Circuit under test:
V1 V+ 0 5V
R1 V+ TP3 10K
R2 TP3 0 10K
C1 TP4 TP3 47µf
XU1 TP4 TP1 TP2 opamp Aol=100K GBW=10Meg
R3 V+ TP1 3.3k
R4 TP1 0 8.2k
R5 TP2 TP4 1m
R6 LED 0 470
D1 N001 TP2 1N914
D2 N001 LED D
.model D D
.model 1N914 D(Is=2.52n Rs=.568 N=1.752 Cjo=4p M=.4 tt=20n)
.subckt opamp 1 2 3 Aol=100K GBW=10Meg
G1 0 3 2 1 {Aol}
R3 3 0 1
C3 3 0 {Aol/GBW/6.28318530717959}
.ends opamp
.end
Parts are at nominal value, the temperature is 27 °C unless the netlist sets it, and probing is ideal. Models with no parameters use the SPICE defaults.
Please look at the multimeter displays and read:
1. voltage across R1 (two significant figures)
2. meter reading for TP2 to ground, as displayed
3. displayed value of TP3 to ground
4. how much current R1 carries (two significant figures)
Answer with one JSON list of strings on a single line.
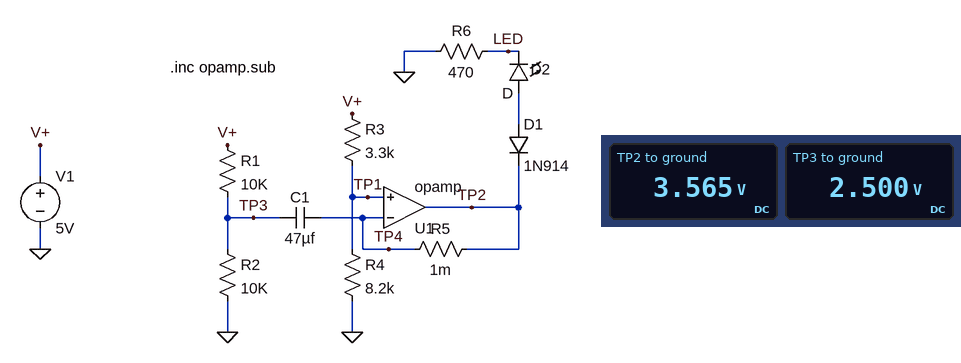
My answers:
["2.5 V", "3.565 V", "2.500 V", "250 µA"]
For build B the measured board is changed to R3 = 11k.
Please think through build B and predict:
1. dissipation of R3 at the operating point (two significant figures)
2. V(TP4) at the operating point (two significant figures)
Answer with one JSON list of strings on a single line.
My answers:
["750 µW", "2.1 V"]
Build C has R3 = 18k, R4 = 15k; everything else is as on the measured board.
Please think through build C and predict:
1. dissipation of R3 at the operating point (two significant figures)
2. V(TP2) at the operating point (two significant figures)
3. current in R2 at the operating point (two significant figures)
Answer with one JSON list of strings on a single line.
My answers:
["410 µW", "2.3 V", "250 µA"]
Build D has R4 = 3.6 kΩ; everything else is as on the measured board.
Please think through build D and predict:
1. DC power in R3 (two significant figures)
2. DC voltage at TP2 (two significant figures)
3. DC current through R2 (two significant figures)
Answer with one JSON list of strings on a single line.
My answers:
["1.7 mW", "2.6 V", "250 µA"]
